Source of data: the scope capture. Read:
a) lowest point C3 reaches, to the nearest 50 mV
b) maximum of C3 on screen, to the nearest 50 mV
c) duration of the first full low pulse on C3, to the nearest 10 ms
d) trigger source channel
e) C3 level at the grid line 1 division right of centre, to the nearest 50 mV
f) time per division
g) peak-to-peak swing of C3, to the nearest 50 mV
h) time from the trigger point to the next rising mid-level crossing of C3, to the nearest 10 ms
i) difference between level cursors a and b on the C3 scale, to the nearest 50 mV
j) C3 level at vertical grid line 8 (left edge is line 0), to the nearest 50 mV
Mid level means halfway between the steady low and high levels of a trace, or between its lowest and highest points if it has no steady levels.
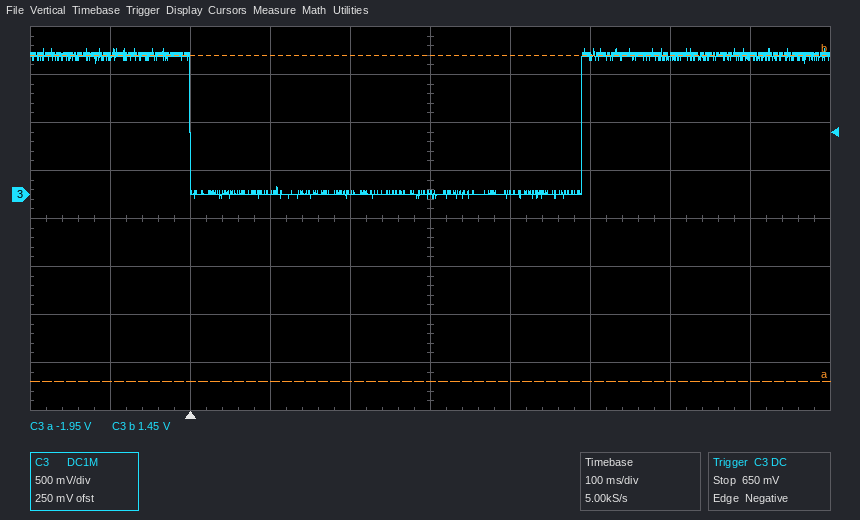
-50 mV
1.50 V
490 ms
C3
0 mV
100 ms
1.55 V
490 ms
3.40 V
1.45 V
